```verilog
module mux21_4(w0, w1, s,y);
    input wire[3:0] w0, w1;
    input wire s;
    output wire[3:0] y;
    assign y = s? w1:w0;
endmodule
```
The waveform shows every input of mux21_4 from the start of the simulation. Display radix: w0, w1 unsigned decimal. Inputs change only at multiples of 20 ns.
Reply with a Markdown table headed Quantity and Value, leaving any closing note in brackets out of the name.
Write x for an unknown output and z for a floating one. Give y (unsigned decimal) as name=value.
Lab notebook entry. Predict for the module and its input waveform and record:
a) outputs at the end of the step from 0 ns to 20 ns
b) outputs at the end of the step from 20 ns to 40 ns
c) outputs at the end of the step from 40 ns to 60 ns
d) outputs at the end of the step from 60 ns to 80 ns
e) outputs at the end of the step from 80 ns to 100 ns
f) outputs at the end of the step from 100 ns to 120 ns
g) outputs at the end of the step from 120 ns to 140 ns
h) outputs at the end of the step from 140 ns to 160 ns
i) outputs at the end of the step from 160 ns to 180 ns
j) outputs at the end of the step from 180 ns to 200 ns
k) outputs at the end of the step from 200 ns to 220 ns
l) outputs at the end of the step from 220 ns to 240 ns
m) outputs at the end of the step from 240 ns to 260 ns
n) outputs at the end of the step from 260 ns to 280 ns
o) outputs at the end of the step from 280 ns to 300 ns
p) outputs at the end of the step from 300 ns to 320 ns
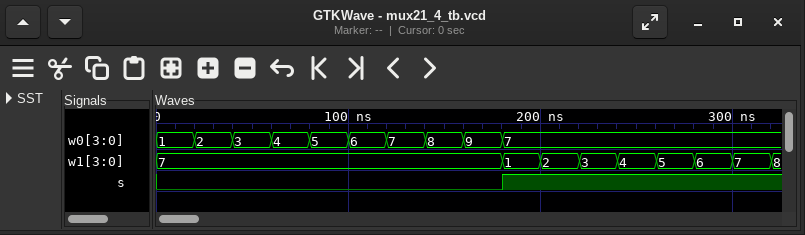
| Quantity | Value |
|---|---|
| outputs at the end of the step from 0 ns to 20 ns | y=1 |
| outputs at the end of the step from 20 ns to 40 ns | y=2 |
| outputs at the end of the step from 40 ns to 60 ns | y=3 |
| outputs at the end of the step from 60 ns to 80 ns | y=4 |
| outputs at the end of the step from 80 ns to 100 ns | y=5 |
| outputs at the end of the step from 100 ns to 120 ns | y=6 |
| outputs at the end of the step from 120 ns to 140 ns | y=7 |
| outputs at the end of the step from 140 ns to 160 ns | y=8 |
| outputs at the end of the step from 160 ns to 180 ns | y=9 |
| outputs at the end of the step from 180 ns to 200 ns | y=1 |
| outputs at the end of the step from 200 ns to 220 ns | y=2 |
| outputs at the end of the step from 220 ns to 240 ns | y=3 |
| outputs at the end of the step from 240 ns to 260 ns | y=4 |
| outputs at the end of the step from 260 ns to 280 ns | y=5 |
| outputs at the end of the step from 280 ns to 300 ns | y=6 |
| outputs at the end of the step from 300 ns to 320 ns | y=7 |
